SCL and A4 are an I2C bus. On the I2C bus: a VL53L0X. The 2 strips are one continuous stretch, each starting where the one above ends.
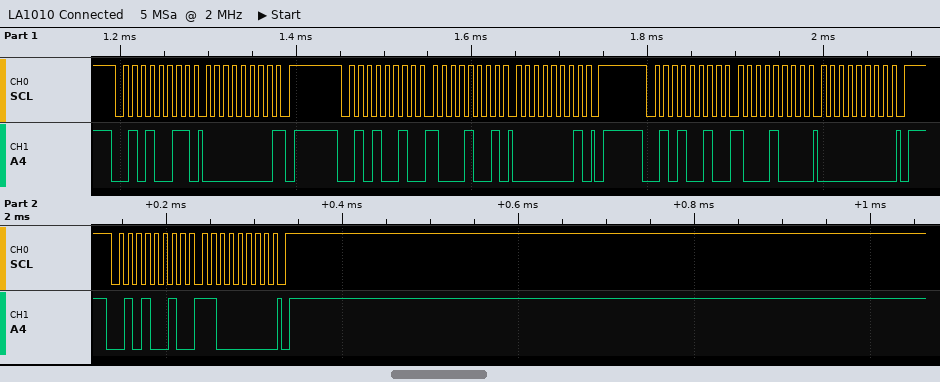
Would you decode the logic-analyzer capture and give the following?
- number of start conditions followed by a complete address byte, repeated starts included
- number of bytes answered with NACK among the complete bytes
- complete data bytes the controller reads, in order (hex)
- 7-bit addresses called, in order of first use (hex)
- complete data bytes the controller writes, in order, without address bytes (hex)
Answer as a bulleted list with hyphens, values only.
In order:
- 4
- 1
- 00
- 0x29
- 89 01 88 00 C0
